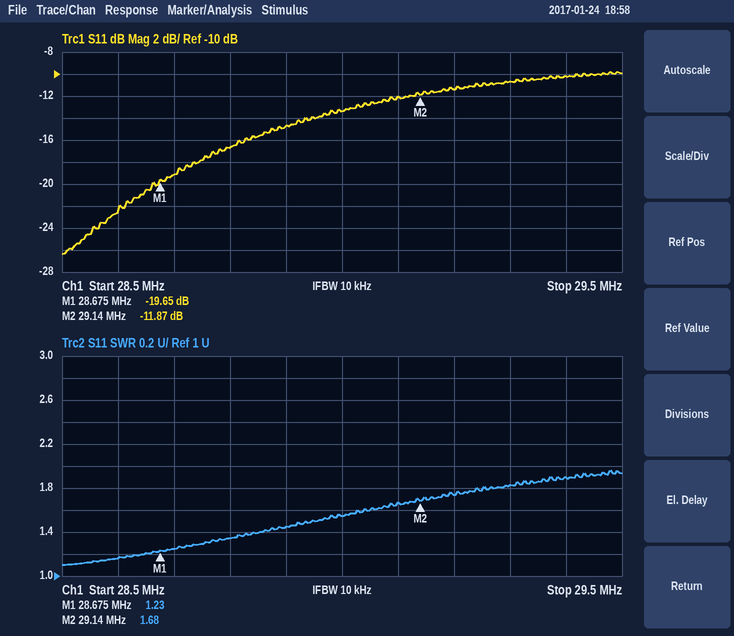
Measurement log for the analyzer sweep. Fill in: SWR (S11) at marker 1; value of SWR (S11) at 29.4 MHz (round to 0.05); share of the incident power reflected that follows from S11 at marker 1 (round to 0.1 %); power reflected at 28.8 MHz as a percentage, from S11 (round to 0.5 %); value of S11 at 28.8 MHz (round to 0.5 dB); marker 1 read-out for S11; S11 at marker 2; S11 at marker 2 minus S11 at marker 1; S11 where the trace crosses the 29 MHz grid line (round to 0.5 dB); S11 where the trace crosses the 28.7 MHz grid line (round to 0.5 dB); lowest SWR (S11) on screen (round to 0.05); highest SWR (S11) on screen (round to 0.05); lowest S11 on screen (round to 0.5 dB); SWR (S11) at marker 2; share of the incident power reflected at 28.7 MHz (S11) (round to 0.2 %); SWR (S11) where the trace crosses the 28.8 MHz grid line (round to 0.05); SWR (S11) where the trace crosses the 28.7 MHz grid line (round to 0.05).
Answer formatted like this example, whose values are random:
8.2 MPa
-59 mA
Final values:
1.23
1.90
1.1 %
2.0 %
-16.5 dB
-19.65 dB
-11.87 dB
7.78 dB
-13.5 dB
-19.0 dB
1.10
1.95
-26.5 dB
1.68
1.2 %
1.35
1.25
